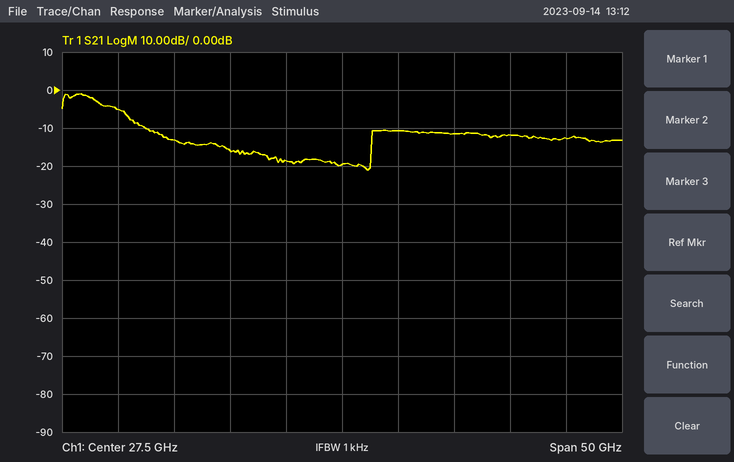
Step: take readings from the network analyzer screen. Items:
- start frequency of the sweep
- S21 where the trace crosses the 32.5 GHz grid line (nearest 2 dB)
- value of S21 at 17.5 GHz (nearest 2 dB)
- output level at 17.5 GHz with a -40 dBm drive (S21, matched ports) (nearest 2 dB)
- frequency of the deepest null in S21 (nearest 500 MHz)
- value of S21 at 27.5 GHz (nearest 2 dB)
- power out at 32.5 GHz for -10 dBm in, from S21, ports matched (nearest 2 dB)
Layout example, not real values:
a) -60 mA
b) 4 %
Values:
a) 2.5 GHz
b) -10 dB
c) -16 dB
d) -56 dBm
e) 30.0 GHz
f) -20 dB
g) -20 dBm
